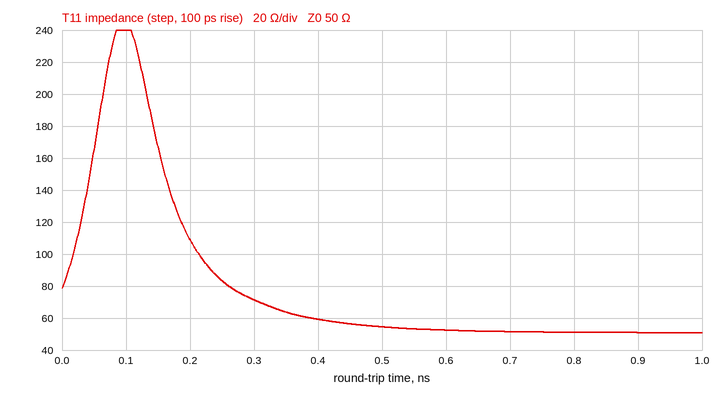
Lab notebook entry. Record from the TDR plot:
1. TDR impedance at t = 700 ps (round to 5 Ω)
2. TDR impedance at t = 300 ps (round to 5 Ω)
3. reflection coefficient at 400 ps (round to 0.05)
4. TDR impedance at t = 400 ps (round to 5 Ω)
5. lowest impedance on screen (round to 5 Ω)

50 Ω
70 Ω
+0.10
60 Ω
50 Ω
